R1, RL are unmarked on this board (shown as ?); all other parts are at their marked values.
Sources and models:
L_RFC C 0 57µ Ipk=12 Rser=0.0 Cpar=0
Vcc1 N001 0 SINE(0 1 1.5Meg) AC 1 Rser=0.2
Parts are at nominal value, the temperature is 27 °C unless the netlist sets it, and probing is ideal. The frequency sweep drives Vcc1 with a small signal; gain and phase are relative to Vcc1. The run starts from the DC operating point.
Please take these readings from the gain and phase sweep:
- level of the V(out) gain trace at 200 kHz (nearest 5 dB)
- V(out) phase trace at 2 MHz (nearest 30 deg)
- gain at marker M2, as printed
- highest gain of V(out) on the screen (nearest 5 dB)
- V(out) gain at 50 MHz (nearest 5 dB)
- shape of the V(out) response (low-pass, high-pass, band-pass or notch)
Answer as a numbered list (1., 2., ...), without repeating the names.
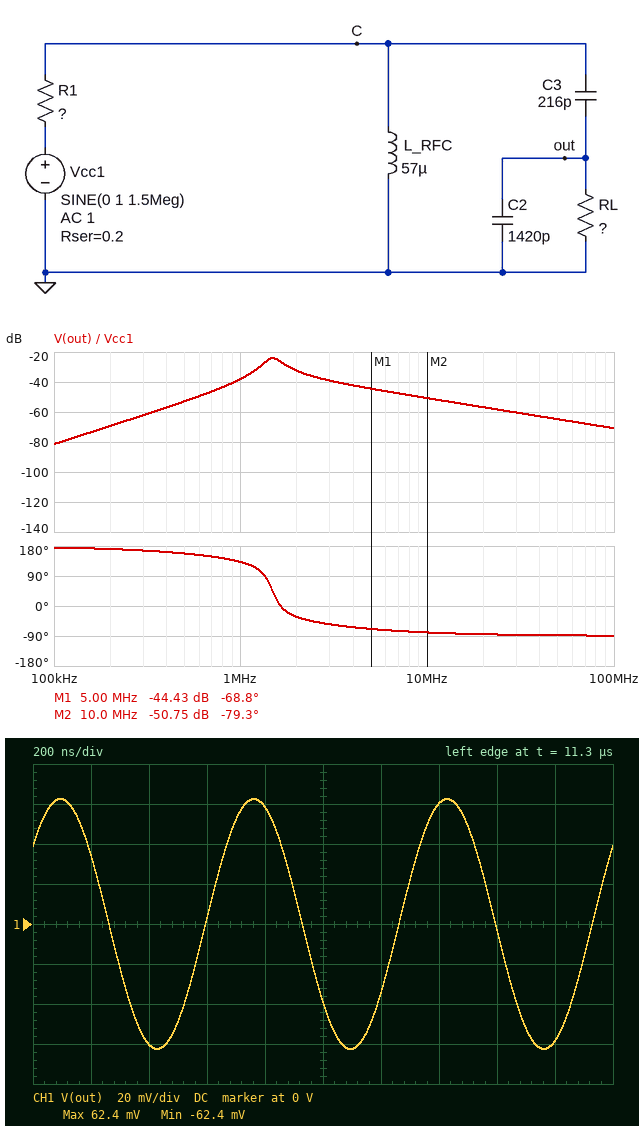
1. -70 dB
2. -30 deg
3. -50.75 dB
4. -25 dB
5. -65 dB
6. band-pass
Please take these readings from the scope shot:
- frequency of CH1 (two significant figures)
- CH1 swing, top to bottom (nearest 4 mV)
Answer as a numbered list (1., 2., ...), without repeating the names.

1. 1.5 MHz
2. 124 mV
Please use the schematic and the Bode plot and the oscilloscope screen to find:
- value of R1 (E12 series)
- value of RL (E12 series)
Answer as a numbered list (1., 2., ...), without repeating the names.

1. 3.9 kΩ
2. 68 Ω
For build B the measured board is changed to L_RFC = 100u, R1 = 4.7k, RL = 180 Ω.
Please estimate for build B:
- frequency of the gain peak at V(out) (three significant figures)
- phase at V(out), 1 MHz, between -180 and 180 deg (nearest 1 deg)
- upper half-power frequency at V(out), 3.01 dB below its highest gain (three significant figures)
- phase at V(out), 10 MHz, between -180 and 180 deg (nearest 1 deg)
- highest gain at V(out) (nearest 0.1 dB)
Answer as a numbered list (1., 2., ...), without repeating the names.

1. 1.15 MHz
2. 81 deg
3. 1.28 MHz
4. -85 deg
5. -21.2 dB
